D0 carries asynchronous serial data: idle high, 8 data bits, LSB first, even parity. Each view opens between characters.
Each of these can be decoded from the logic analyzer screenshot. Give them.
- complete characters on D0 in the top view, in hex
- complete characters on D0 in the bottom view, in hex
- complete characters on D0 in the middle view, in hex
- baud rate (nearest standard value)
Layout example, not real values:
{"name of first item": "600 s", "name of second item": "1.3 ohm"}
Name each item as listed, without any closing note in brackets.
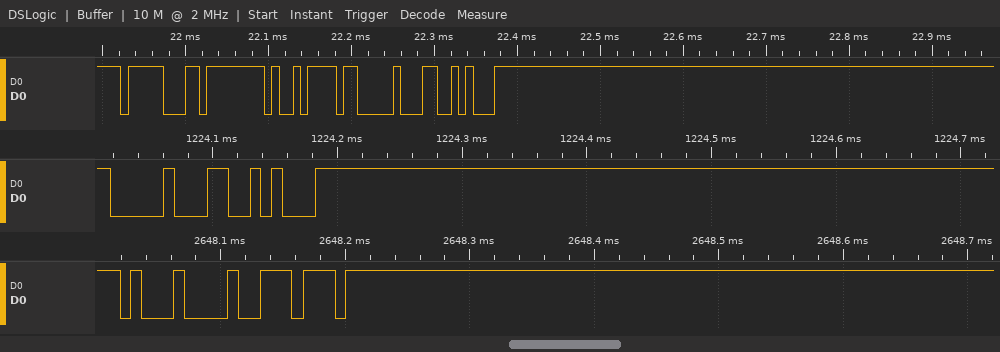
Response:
{"complete characters on D0 in the top view, in hex": "1F, FF, 7A, 10, 8A", "complete characters on D0 in the bottom view, in hex": "11, EE", "complete characters on D0 in the middle view, in hex": "10, 8A", "baud rate": "115200 baud"}
